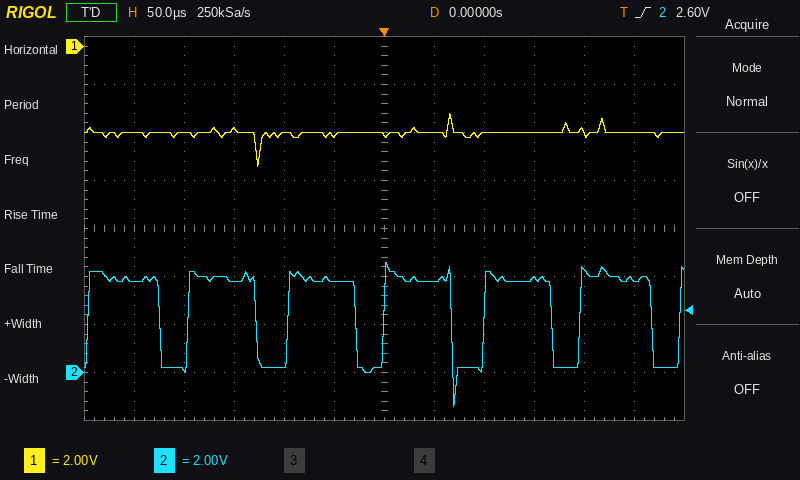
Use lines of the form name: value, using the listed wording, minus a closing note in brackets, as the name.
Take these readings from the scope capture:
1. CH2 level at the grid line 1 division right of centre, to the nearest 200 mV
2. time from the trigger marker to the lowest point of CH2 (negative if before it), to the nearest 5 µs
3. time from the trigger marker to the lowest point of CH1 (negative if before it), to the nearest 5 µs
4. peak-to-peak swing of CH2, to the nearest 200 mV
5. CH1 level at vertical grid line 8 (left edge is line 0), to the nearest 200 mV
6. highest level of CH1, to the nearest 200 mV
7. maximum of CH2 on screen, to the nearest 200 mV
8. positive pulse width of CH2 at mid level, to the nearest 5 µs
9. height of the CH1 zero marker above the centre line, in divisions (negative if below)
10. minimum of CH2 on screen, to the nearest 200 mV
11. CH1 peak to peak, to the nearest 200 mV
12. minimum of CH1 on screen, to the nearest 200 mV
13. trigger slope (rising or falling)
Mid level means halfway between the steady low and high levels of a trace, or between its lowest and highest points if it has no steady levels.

CH2 level at the grid line 1 division right of centre, to the nearest 200 mV: 3.8 V
time from the trigger marker to the lowest point of CH2 (negative if before it), to the nearest 5 µs: +70 µs
time from the trigger marker to the lowest point of CH1 (negative if before it), to the nearest 5 µs: -125 µs
peak-to-peak swing of CH2, to the nearest 200 mV: 6.0 V
CH1 level at vertical grid line 8 (left edge is line 0), to the nearest 200 mV: -3.6 V
highest level of CH1, to the nearest 200 mV: -2.8 V
maximum of CH2 on screen, to the nearest 200 mV: 4.6 V
positive pulse width of CH2 at mid level, to the nearest 5 µs: 70 µs
height of the CH1 zero marker above the centre line, in divisions: +3.8 div
minimum of CH2 on screen, to the nearest 200 mV: -1.4 V
CH1 peak to peak, to the nearest 200 mV: 2.2 V
minimum of CH1 on screen, to the nearest 200 mV: -5.0 V
trigger slope: rising
